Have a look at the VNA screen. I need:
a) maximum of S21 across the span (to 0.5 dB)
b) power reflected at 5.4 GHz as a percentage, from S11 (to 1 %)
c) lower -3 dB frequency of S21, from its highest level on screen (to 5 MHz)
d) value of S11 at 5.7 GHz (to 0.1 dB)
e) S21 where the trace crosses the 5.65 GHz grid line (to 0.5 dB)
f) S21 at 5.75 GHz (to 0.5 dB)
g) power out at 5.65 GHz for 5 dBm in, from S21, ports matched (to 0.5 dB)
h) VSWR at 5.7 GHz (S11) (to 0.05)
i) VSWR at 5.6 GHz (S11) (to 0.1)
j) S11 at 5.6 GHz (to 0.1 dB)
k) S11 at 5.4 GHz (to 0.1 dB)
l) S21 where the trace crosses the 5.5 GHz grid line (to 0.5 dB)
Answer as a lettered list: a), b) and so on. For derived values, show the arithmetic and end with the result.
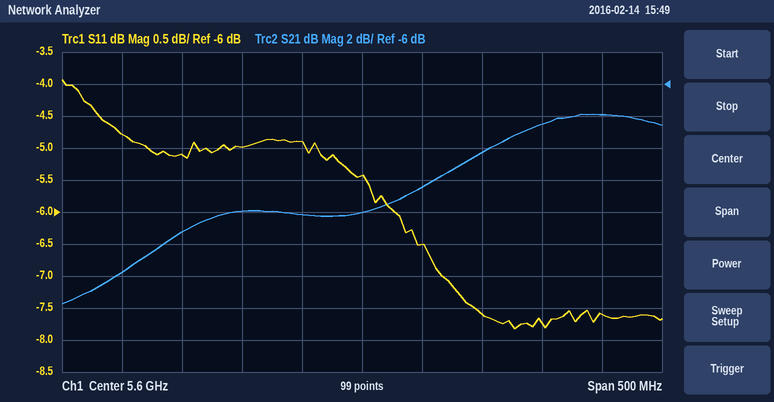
a) -8.0 dB
b) 10^(-4.8/10) ≈ 33 %
c) 5.685 GHz
d) -7.6 dB
e) -12.5 dB
f) -8.5 dB
g) 5 dBm + (-12.5 dB) = -7.5 dBm
h) |Γ| = 10^(-7.6/20) = 0.4169; VSWR = (1 + 0.4169)/(1 − 0.4169) ≈ 2.43, so 2.45 to the nearest 0.05
i) |Γ| = 10^(-5.4/20) = 0.5370; VSWR = (1 + 0.5370)/(1 − 0.5370) ≈ 3.3
j) -5.4 dB
k) -4.8 dB
l) -14.0 dB
